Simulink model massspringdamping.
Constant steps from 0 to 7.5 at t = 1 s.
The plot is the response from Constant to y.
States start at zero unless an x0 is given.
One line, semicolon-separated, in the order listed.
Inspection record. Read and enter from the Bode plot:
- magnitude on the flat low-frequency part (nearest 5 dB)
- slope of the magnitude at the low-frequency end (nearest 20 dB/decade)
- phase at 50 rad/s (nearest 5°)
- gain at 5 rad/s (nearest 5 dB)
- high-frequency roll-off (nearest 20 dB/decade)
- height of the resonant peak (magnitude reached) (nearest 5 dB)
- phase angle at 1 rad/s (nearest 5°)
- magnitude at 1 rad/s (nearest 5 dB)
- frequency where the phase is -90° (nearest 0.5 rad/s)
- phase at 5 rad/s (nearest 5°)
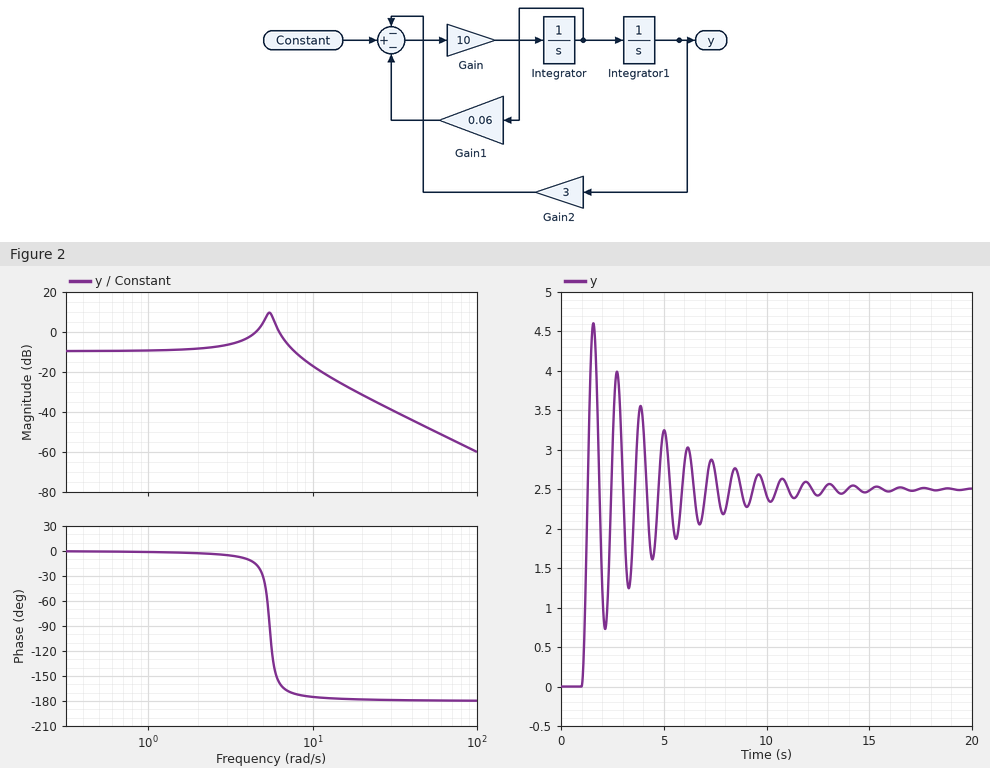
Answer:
-10 dB; 0 dB/decade; -180°; 5 dB; -40 dB/decade; 10 dB; 0°; -10 dB; 5.5 rad/s; -30°
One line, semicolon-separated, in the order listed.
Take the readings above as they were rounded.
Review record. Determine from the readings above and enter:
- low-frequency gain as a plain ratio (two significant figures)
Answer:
0.32
